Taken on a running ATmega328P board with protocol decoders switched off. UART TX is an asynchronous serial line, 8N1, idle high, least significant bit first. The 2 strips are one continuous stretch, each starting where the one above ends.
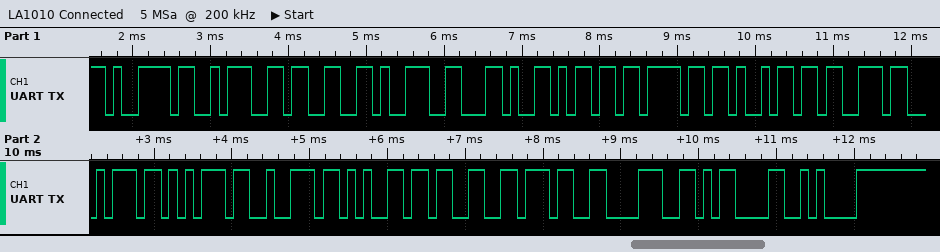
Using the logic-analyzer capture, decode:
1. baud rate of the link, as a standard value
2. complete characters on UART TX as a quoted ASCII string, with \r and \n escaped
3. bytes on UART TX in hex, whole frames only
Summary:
9600 baud
"y:39,moisture378\r\n"
79 3A 33 39 2C 6D 6F 69 73 74 75 72 65 33 37 38 0D 0A
